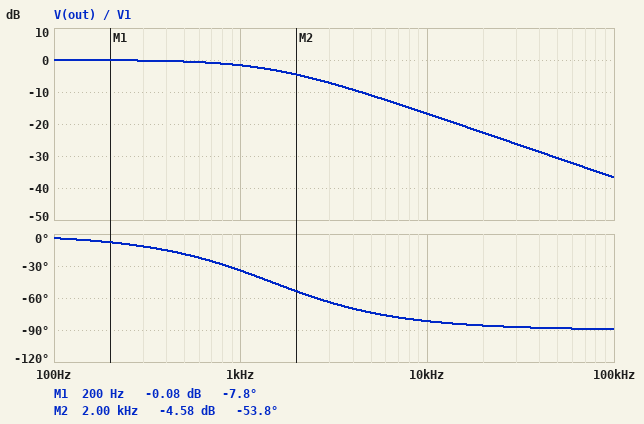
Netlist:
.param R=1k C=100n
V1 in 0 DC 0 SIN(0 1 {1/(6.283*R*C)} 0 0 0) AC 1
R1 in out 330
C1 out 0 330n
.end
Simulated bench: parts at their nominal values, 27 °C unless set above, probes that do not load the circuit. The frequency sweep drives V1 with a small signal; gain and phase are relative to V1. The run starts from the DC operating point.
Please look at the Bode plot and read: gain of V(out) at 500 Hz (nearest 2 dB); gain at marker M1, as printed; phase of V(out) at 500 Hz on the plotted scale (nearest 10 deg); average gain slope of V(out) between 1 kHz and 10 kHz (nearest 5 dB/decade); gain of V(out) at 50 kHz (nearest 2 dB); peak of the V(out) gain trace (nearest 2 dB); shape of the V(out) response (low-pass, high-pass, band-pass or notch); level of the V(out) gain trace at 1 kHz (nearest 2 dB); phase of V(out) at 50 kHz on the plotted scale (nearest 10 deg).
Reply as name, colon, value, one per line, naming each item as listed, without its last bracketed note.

gain of V(out) at 500 Hz: 0 dB
gain at marker M1, as printed: -0.08 dB
phase of V(out) at 500 Hz on the plotted scale: -20 deg
average gain slope of V(out) between 1 kHz and 10 kHz: -15 dB/decade
gain of V(out) at 50 kHz: -30 dB
peak of the V(out) gain trace: 0 dB
shape of the V(out) response: low-pass
level of the V(out) gain trace at 1 kHz: -2 dB
phase of V(out) at 50 kHz on the plotted scale: -90 deg
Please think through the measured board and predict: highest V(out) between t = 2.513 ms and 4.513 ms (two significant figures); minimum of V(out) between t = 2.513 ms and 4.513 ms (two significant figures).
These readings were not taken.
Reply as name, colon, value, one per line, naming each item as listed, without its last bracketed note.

highest V(out) between t = 2.513 ms and 4.513 ms: 680 mV
minimum of V(out) between t = 2.513 ms and 4.513 ms: -680 mV
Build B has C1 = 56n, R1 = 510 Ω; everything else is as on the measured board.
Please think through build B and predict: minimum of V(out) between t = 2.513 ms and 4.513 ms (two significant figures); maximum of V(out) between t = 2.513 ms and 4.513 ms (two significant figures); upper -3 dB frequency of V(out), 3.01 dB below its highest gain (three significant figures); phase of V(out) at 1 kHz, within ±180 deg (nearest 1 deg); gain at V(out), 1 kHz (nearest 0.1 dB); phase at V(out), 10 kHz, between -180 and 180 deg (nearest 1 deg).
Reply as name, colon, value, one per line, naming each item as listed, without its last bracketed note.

minimum of V(out) between t = 2.513 ms and 4.513 ms: -960 mV
maximum of V(out) between t = 2.513 ms and 4.513 ms: 960 mV
upper -3 dB frequency of V(out), 3.01 dB below its highest gain: 5.57 kHz
phase of V(out) at 1 kHz, within ±180 deg: -10 deg
gain at V(out), 1 kHz: -0.1 dB
phase at V(out), 10 kHz, between -180 and 180 deg: -61 deg
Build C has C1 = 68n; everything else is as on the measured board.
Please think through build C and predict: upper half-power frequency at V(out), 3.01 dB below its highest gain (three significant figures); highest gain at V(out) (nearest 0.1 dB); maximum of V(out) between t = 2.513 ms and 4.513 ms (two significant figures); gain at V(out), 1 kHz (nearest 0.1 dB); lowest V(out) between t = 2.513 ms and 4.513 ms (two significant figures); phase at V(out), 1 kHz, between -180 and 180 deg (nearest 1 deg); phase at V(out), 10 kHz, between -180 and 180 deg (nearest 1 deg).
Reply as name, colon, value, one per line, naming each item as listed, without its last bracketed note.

upper half-power frequency at V(out), 3.01 dB below its highest gain: 7.09 kHz
highest gain at V(out): 0 dB
maximum of V(out) between t = 2.513 ms and 4.513 ms: 980 mV
gain at V(out), 1 kHz: -0.1 dB
lowest V(out) between t = 2.513 ms and 4.513 ms: -980 mV
phase at V(out), 1 kHz, between -180 and 180 deg: -8 deg
phase at V(out), 10 kHz, between -180 and 180 deg: -55 deg
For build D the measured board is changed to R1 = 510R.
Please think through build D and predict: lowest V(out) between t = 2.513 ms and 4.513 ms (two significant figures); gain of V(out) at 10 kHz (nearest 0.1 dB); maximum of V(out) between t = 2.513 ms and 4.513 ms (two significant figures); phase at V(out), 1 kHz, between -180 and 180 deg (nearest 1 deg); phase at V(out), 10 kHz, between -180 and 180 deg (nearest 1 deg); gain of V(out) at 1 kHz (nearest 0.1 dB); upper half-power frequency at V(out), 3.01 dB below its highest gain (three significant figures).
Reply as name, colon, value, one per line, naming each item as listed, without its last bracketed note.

lowest V(out) between t = 2.513 ms and 4.513 ms: -510 mV
gain of V(out) at 10 kHz: -20.5 dB
maximum of V(out) between t = 2.513 ms and 4.513 ms: 510 mV
phase at V(out), 1 kHz, between -180 and 180 deg: -47 deg
phase at V(out), 10 kHz, between -180 and 180 deg: -85 deg
gain of V(out) at 1 kHz: -3.3 dB
upper half-power frequency at V(out), 3.01 dB below its highest gain: 946 Hz
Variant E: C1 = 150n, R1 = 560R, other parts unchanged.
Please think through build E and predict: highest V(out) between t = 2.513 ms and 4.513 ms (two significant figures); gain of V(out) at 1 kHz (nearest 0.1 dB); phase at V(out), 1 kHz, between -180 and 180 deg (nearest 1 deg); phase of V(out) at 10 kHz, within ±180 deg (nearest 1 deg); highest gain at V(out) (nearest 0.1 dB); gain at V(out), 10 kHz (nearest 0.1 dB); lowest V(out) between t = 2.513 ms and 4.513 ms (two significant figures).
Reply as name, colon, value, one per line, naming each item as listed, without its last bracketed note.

highest V(out) between t = 2.513 ms and 4.513 ms: 770 mV
gain of V(out) at 1 kHz: -1.1 dB
phase at V(out), 1 kHz, between -180 and 180 deg: -28 deg
phase of V(out) at 10 kHz, within ±180 deg: -79 deg
highest gain at V(out): 0 dB
gain at V(out), 10 kHz: -14.6 dB
lowest V(out) between t = 2.513 ms and 4.513 ms: -770 mV
